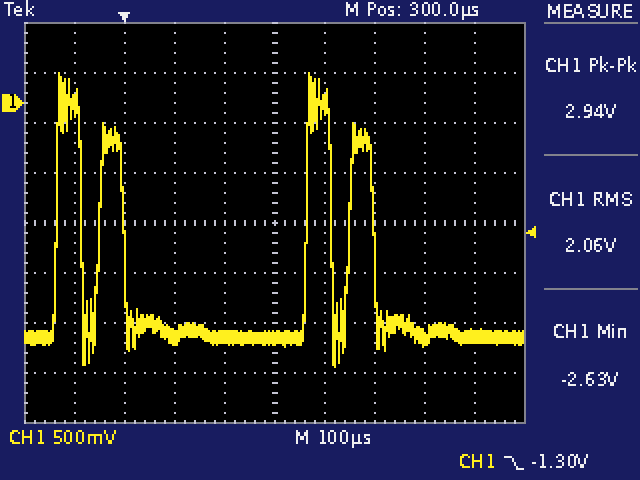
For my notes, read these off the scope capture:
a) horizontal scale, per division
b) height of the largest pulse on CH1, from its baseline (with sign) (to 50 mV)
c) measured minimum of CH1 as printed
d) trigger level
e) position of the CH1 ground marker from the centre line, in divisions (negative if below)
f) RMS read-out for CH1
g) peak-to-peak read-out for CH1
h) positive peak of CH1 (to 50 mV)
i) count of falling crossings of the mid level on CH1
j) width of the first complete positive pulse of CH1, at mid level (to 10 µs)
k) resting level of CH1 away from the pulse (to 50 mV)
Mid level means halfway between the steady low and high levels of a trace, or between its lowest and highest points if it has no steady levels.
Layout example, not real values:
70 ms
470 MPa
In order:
100 µs
+2.65 V
-2.63 V
-1.30 V
+2.4 div
2.06 V
2.94 V
300 mV
4
50 µs
-2.35 V
